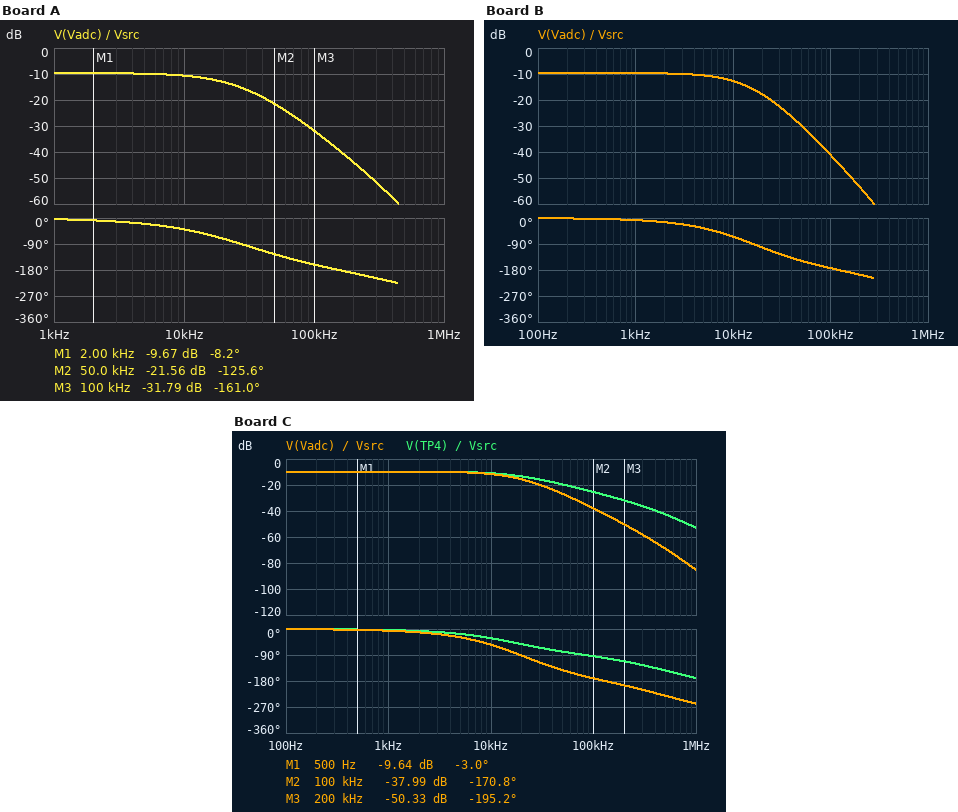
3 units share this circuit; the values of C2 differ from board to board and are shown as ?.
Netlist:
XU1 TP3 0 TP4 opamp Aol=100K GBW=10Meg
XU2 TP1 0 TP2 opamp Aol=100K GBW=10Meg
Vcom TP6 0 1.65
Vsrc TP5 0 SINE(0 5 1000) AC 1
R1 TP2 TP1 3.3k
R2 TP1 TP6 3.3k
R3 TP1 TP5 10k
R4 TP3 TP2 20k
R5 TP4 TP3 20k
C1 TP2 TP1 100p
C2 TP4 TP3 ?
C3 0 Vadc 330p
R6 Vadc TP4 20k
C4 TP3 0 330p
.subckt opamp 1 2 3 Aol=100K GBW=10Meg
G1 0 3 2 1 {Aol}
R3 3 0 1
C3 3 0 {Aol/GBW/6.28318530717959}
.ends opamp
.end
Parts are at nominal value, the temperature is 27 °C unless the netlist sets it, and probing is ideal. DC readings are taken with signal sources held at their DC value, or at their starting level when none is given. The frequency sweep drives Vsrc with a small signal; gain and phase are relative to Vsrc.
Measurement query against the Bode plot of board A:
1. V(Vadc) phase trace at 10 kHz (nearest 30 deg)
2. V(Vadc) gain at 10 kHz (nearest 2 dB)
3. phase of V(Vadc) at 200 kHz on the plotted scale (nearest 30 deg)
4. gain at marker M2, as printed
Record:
-30 deg
-10 dB
-180 deg
-21.56 dB
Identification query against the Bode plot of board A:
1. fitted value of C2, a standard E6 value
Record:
220 pF
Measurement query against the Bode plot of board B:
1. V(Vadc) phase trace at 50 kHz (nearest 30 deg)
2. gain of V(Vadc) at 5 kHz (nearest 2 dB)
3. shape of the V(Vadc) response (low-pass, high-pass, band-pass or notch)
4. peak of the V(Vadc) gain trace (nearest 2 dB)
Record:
-150 deg
-10 dB
low-pass
-10 dB
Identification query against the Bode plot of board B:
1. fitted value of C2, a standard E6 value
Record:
680 pF
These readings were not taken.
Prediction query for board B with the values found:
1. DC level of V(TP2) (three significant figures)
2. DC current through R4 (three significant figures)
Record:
-1.65 V
82.5 µA
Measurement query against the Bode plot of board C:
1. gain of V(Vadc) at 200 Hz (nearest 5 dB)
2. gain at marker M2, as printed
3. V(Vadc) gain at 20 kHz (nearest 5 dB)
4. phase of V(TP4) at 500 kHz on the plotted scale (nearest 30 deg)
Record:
-10 dB
-37.99 dB
-15 dB
-150 deg
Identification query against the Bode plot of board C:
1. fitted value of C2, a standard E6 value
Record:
470 pF
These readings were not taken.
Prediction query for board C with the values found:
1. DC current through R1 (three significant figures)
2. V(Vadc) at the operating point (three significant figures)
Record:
500 µA
1.65 V
